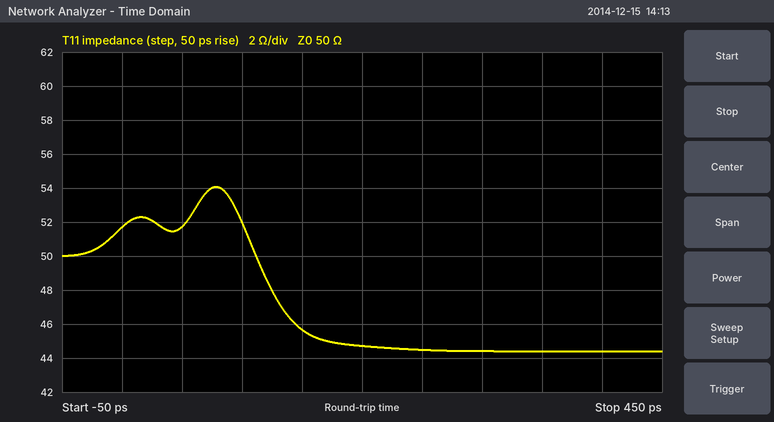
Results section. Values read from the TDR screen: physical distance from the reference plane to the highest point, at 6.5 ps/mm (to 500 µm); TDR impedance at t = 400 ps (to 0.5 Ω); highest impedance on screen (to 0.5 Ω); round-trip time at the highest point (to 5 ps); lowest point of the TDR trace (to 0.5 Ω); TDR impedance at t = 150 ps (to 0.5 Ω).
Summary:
6.0 mm
44.5 Ω
54.0 Ω
80 ps
44.5 Ω
45.5 Ω
